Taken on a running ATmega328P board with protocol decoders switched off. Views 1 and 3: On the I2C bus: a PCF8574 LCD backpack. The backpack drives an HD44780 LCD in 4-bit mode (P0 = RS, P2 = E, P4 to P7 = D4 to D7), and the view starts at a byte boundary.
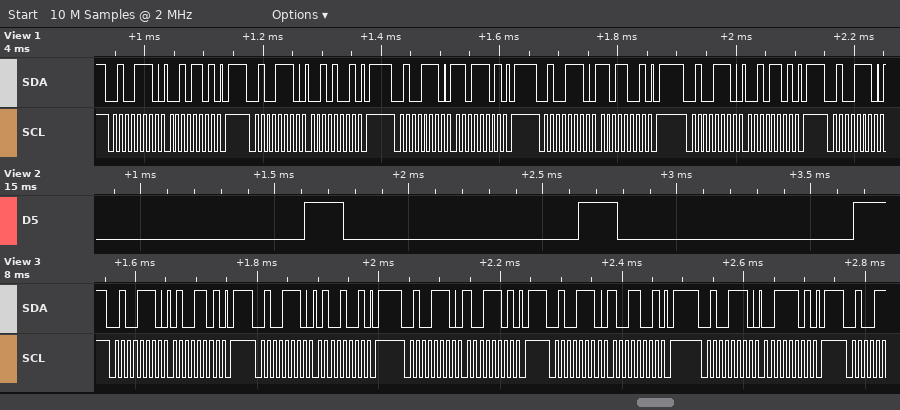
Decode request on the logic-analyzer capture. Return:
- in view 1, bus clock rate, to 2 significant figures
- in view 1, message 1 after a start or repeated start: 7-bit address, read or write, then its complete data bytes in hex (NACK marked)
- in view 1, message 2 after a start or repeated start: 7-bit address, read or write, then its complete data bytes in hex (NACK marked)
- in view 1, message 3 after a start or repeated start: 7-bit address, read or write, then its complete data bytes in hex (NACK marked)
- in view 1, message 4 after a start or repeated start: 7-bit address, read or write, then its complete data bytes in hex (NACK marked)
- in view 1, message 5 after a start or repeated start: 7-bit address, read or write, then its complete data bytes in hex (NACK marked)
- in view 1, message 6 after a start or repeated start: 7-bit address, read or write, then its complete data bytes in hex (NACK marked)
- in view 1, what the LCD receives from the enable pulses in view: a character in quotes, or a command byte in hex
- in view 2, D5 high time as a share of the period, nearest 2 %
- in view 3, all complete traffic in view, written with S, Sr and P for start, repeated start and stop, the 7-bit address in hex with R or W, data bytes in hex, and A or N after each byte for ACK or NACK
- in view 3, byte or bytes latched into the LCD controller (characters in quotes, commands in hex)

100 kHz
0x27 write: 2D
0x27 write: 29
0x27 write: DD
0x27 write: D9
0x27 write: 2D
0x27 write
'-'
14 %
S 27W A 4D A P S 27W A 49 A P S 27W A 9D A P S 27W A 99 A P S 27W A 3D A P
'I'
